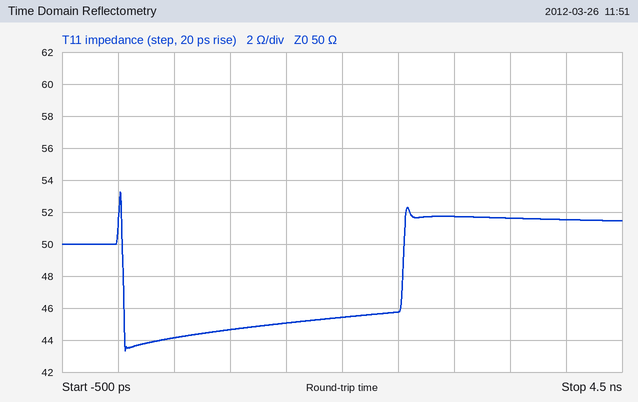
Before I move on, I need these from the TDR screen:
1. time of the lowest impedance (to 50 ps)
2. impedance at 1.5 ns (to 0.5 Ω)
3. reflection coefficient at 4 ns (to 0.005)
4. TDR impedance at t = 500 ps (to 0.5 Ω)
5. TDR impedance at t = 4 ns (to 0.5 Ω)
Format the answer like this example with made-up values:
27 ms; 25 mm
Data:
50 ps; 45.0 Ω; +0.015; 44.0 Ω; 51.5 Ω
